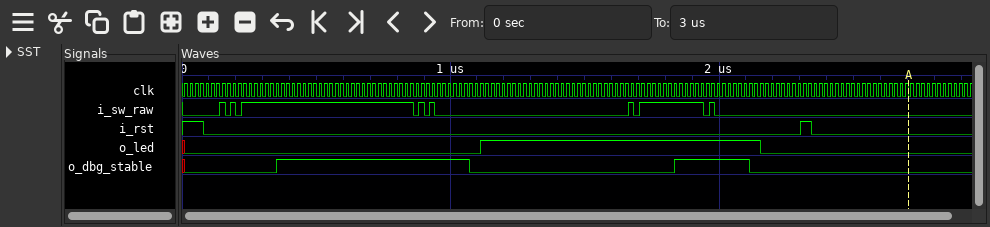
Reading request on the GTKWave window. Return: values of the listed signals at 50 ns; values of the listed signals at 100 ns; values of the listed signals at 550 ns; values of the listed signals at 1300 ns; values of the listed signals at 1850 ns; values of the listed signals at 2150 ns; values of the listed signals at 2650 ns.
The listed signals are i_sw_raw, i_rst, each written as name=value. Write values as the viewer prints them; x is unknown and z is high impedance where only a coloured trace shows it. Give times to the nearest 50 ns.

i_sw_raw=0, i_rst=1
i_sw_raw=0, i_rst=0
i_sw_raw=1, i_rst=0
i_sw_raw=0, i_rst=0
i_sw_raw=1, i_rst=0
i_sw_raw=0, i_rst=0
i_sw_raw=0, i_rst=0
